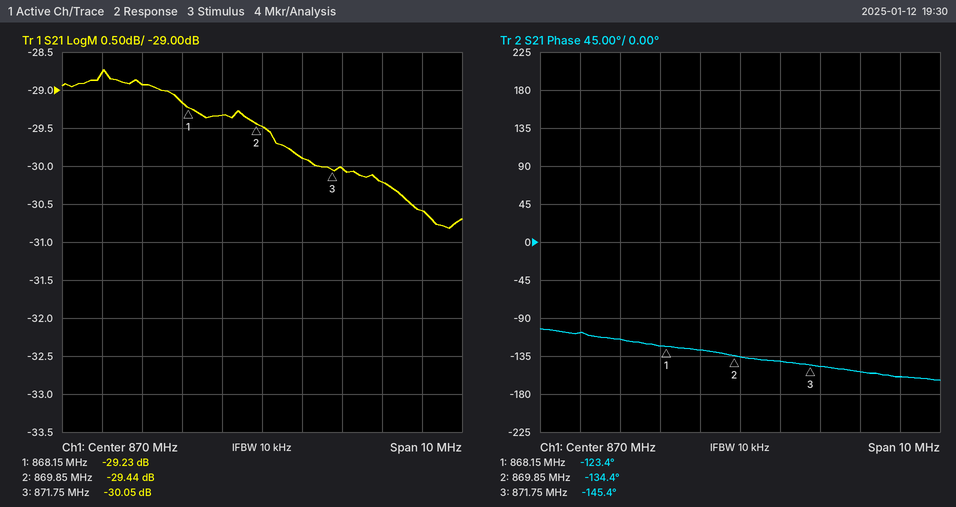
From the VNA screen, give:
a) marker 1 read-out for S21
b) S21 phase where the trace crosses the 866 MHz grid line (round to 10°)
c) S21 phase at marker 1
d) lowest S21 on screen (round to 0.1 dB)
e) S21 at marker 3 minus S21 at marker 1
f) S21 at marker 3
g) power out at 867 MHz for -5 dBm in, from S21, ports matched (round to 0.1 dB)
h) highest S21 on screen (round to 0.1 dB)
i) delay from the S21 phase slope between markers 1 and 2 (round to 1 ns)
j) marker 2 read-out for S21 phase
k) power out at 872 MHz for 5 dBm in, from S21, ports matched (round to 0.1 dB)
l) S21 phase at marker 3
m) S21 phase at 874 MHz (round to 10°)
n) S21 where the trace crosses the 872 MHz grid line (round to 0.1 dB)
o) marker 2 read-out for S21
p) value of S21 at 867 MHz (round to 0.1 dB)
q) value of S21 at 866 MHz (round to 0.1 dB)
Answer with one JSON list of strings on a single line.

["-29.23 dB", "-110°", "-123.4°", "-30.8 dB", "-0.82 dB", "-30.05 dB", "-33.9 dBm", "-28.7 dB", "18 ns", "-134.4°", "-25.0 dBm", "-145.4°", "-160°", "-30.0 dB", "-29.44 dB", "-28.9 dB", "-28.8 dB"]
